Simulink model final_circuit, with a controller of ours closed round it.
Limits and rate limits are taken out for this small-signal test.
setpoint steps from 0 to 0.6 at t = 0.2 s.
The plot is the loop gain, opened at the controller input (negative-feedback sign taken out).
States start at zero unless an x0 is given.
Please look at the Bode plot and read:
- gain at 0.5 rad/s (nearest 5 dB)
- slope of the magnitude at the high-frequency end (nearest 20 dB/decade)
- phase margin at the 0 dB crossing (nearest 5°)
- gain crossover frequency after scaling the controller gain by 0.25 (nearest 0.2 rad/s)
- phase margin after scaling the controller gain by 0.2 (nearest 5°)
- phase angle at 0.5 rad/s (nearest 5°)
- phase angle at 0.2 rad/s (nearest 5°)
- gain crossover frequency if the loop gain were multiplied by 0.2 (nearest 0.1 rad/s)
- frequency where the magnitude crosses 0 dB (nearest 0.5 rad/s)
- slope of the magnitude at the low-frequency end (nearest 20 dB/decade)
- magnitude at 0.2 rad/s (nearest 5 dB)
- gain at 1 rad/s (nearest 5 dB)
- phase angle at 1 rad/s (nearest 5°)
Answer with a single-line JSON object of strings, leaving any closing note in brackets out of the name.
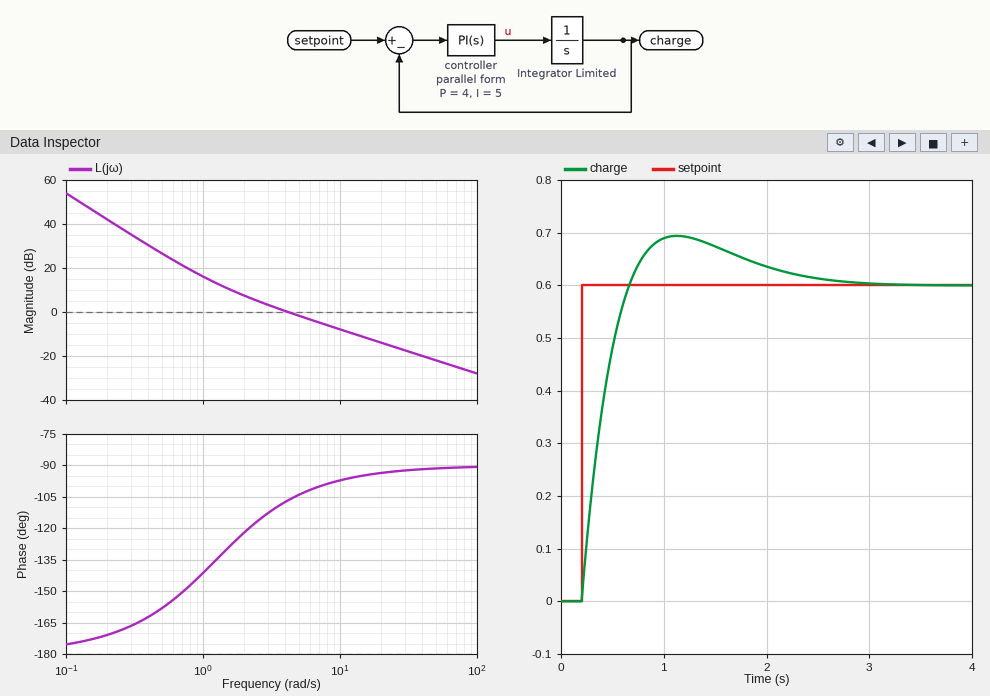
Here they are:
{"gain at 0.5 rad/s": "25 dB", "slope of the magnitude at the high-frequency end": "-20 dB/decade", "phase margin at the 0 dB crossing": "75°", "gain crossover frequency after scaling the controller gain by 0.25": "1.4 rad/s", "phase margin after scaling the controller gain by 0.2": "45°", "phase angle at 0.5 rad/s": "-160°", "phase angle at 0.2 rad/s": "-170°", "gain crossover frequency if the loop gain were multiplied by 0.2": "1.2 rad/s", "frequency where the magnitude crosses 0 dB": "4.0 rad/s", "slope of the magnitude at the low-frequency end": "-40 dB/decade", "magnitude at 0.2 rad/s": "40 dB", "gain at 1 rad/s": "15 dB", "phase angle at 1 rad/s": "-140°"}
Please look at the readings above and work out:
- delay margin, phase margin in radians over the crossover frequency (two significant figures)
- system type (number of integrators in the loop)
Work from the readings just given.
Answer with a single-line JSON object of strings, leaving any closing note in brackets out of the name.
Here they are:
{"delay margin, phase margin in radians over the crossover frequency": "0.33 s", "system type": "2"}
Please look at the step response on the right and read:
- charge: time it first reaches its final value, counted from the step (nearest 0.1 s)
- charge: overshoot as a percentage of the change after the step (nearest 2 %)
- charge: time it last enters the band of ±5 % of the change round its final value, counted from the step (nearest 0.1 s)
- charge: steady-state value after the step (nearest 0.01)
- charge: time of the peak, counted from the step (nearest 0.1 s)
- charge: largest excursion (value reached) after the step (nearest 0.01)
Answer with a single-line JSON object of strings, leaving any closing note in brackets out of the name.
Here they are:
{"charge: time it first reaches its final value, counted from the step": "0.5 s", "charge: overshoot as a percentage of the change after the step": "16 %", "charge: time it last enters the band of ±5 % of the change round its final value, counted from the step": "1.9 s", "charge: steady-state value after the step": "0.60", "charge: time of the peak, counted from the step": "0.9 s", "charge: largest excursion (value reached) after the step": "0.69"}
